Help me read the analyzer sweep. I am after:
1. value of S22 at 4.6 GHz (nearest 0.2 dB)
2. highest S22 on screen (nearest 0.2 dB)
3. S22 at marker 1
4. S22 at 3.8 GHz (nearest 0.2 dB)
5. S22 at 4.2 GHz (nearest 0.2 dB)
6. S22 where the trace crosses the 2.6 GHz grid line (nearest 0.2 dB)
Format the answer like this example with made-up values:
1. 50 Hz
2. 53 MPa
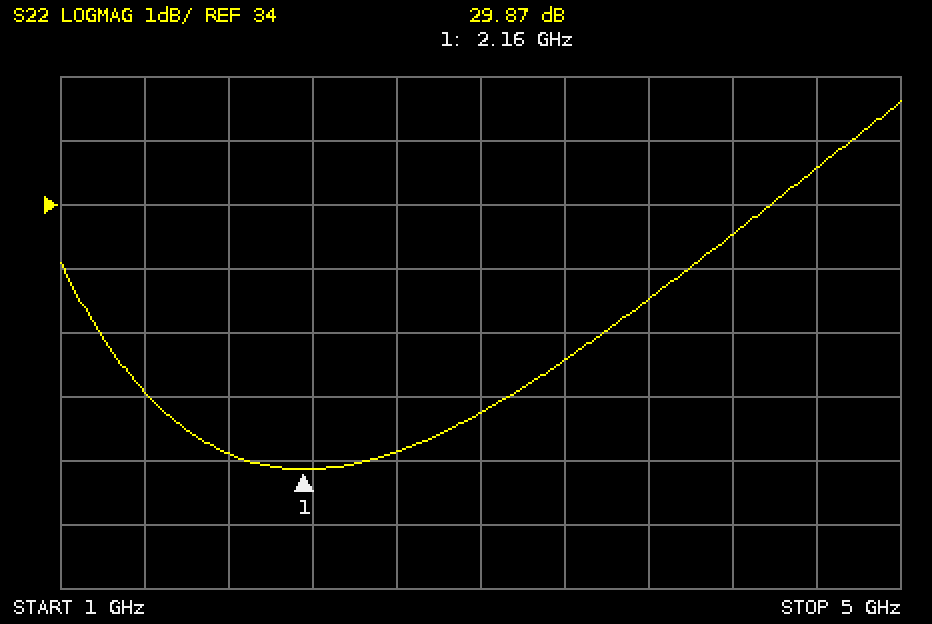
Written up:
1. 34.6 dB
2. 35.6 dB
3. 29.87 dB
4. 32.6 dB
5. 33.6 dB
6. 30.2 dB
